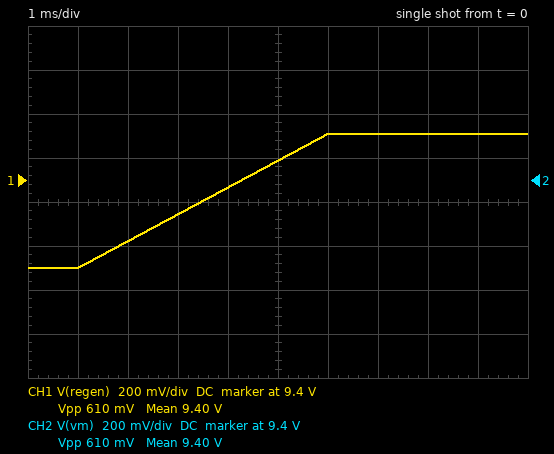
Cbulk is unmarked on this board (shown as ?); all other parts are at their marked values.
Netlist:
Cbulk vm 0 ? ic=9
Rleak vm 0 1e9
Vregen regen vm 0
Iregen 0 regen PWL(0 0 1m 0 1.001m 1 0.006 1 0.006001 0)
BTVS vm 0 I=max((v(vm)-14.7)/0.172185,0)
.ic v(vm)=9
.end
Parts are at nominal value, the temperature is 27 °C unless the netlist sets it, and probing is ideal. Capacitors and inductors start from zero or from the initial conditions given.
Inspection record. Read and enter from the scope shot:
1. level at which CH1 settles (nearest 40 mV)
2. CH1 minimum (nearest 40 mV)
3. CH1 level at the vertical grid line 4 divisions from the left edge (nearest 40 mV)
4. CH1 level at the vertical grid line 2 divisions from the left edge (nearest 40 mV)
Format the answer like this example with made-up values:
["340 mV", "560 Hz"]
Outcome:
["9.60 V", "9.00 V", "9.36 V", "9.12 V"]
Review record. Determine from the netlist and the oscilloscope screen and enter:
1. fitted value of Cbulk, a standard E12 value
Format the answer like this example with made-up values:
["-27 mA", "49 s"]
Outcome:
["8.2 mF"]
